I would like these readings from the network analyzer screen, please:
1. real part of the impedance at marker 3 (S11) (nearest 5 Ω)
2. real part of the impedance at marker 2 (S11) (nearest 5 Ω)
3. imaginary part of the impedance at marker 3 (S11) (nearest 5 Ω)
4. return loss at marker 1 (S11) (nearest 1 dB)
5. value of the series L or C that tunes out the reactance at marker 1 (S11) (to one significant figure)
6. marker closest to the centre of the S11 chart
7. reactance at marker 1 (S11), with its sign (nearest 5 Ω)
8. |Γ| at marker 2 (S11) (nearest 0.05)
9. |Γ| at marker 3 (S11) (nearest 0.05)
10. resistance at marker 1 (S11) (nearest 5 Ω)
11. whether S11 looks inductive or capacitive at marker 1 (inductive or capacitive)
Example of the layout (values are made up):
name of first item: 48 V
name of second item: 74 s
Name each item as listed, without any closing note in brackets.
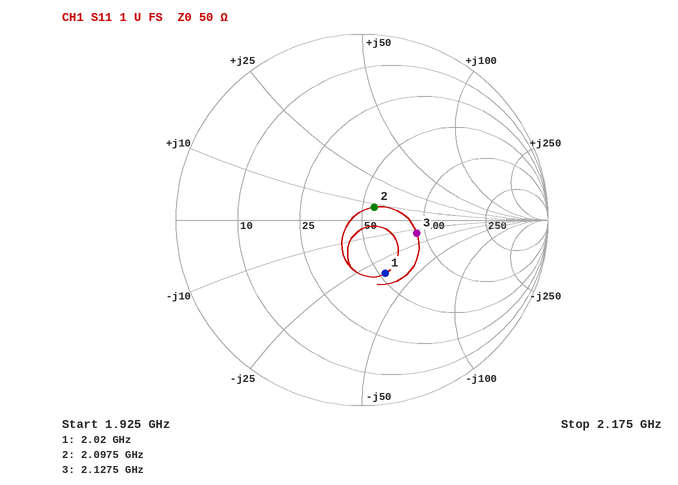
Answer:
real part of the impedance at marker 3 (S11): 90 Ω
real part of the impedance at marker 2 (S11): 55 Ω
imaginary part of the impedance at marker 3 (S11): -15 Ω
return loss at marker 1 (S11): 10 dB
value of the series L or C that tunes out the reactance at marker 1 (S11): 3 nH
marker closest to the centre of the S11 chart: marker 2
reactance at marker 1 (S11), with its sign: -35 Ω
|Γ| at marker 2 (S11): 0.10
|Γ| at marker 3 (S11): 0.30
resistance at marker 1 (S11): 55 Ω
whether S11 looks inductive or capacitive at marker 1: capacitive
